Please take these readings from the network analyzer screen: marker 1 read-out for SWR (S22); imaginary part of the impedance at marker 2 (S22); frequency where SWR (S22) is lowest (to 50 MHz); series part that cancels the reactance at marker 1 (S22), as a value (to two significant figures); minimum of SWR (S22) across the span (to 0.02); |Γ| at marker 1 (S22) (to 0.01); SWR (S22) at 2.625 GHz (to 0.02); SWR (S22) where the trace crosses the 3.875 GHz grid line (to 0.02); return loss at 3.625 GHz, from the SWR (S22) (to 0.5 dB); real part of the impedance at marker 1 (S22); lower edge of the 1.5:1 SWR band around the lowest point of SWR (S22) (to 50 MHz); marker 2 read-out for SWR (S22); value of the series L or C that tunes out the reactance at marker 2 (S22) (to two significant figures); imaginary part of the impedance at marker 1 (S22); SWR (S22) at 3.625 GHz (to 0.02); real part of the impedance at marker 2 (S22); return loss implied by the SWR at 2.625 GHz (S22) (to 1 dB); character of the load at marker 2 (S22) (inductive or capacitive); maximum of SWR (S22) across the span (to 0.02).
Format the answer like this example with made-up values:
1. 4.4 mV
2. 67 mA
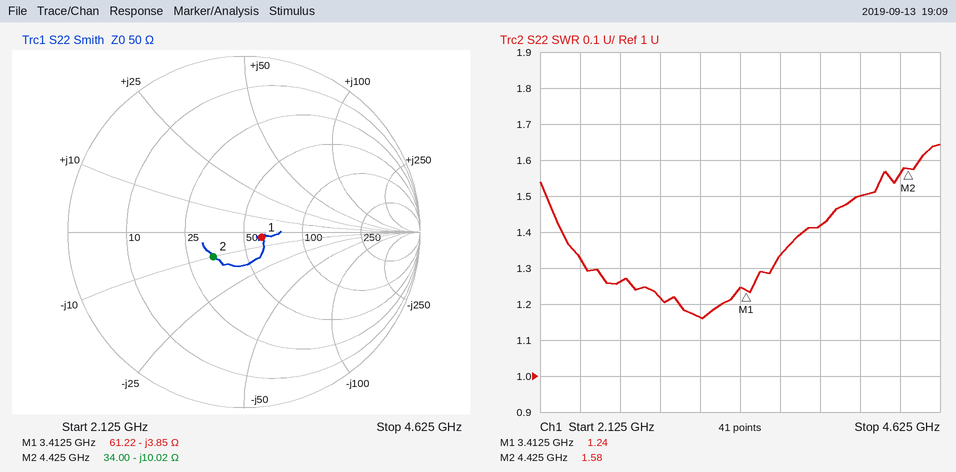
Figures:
1. 1.24
2. -10.02 Ω
3. 3.15 GHz
4. 180 pH
5. 1.16
6. 0.11
7. 1.26
8. 1.42
9. 17.0 dB
10. 61.22 Ω
11. 2.15 GHz
12. 1.58
13. 360 pH
14. -3.85 Ω
15. 1.34
16. 34.00 Ω
17. 19 dB
18. capacitive
19. 1.64
